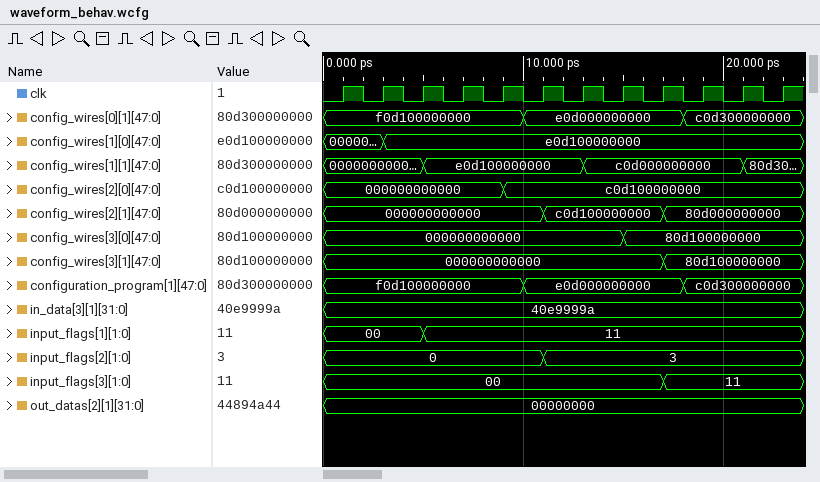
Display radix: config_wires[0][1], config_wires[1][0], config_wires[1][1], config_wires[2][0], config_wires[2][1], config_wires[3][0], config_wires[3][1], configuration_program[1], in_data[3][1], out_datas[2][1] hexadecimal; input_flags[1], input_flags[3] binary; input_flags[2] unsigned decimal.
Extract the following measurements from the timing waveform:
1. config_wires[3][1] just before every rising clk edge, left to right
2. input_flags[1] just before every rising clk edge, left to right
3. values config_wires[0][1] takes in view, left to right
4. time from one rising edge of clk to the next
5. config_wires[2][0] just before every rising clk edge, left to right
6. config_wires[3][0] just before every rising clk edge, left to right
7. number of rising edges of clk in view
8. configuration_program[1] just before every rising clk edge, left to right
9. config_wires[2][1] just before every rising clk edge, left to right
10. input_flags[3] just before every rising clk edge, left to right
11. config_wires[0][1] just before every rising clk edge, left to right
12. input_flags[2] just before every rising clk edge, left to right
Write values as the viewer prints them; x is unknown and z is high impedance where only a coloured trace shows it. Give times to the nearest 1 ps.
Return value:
000000000000, 000000000000, 000000000000, 000000000000, 000000000000, 000000000000, 000000000000, 000000000000, 000000000000, 80d100000000, 80d100000000, 80d100000000
00, 00, 00, 11, 11, 11, 11, 11, 11, 11, 11, 11
f0d100000000, e0d000000000, c0d300000000
2 ps
000000000000, 000000000000, 000000000000, 000000000000, 000000000000, c0d100000000, c0d100000000, c0d100000000, c0d100000000, c0d100000000, c0d100000000, c0d100000000
000000000000, 000000000000, 000000000000, 000000000000, 000000000000, 000000000000, 000000000000, 000000000000, 80d100000000, 80d100000000, 80d100000000, 80d100000000
12
f0d100000000, f0d100000000, f0d100000000, f0d100000000, f0d100000000, e0d000000000, e0d000000000, e0d000000000, e0d000000000, c0d300000000, c0d300000000, c0d300000000
000000000000, 000000000000, 000000000000, 000000000000, 000000000000, 000000000000, c0d100000000, c0d100000000, c0d100000000, 80d000000000, 80d000000000, 80d000000000
00, 00, 00, 00, 00, 00, 00, 00, 00, 11, 11, 11
f0d100000000, f0d100000000, f0d100000000, f0d100000000, f0d100000000, e0d000000000, e0d000000000, e0d000000000, e0d000000000, c0d300000000, c0d300000000, c0d300000000
0, 0, 0, 0, 0, 0, 3, 3, 3, 3, 3, 3
